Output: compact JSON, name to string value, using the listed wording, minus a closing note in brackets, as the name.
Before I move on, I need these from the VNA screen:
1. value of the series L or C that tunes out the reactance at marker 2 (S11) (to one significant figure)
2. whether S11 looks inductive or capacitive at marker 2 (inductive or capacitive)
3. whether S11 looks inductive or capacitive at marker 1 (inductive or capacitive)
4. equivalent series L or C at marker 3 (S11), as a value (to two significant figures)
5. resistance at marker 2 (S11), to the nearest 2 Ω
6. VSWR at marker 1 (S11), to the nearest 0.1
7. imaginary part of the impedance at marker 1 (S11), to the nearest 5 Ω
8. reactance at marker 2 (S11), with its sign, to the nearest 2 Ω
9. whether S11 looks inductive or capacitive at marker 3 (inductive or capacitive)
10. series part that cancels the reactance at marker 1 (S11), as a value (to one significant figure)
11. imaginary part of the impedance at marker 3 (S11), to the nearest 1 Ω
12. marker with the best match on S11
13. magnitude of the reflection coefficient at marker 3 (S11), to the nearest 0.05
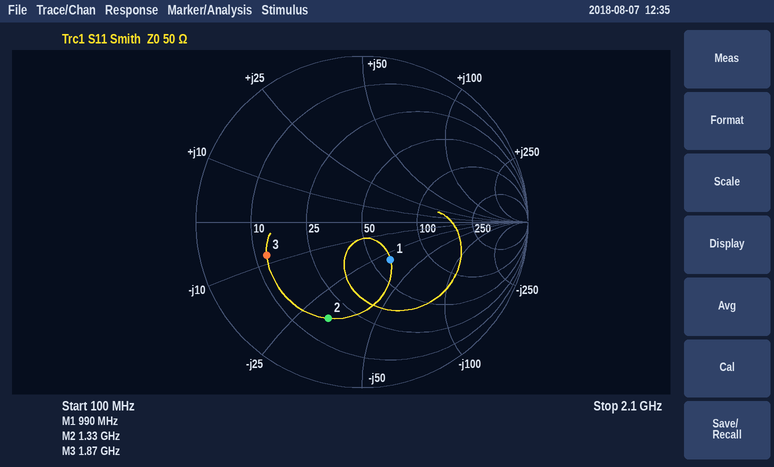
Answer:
{"value of the series L or C that tunes out the reactance at marker 2 (S11)": "4 nH", "whether S11 looks inductive or capacitive at marker 2": "capacitive", "whether S11 looks inductive or capacitive at marker 1": "capacitive", "equivalent series L or C at marker 3 (S11), as a value": "11 pF", "resistance at marker 2 (S11), to the nearest 2 Ω": "18 Ω", "VSWR at marker 1 (S11), to the nearest 0.1": "1.8", "imaginary part of the impedance at marker 1 (S11), to the nearest 5 Ω": "-30 Ω", "reactance at marker 2 (S11), with its sign, to the nearest 2 Ω": "-32 Ω", "whether S11 looks inductive or capacitive at marker 3": "capacitive", "series part that cancels the reactance at marker 1 (S11), as a value": "5 nH", "imaginary part of the impedance at marker 3 (S11), to the nearest 1 Ω": "-8 Ω", "marker with the best match on S11": "marker 1", "magnitude of the reflection coefficient at marker 3 (S11), to the nearest 0.05": "0.60"}
